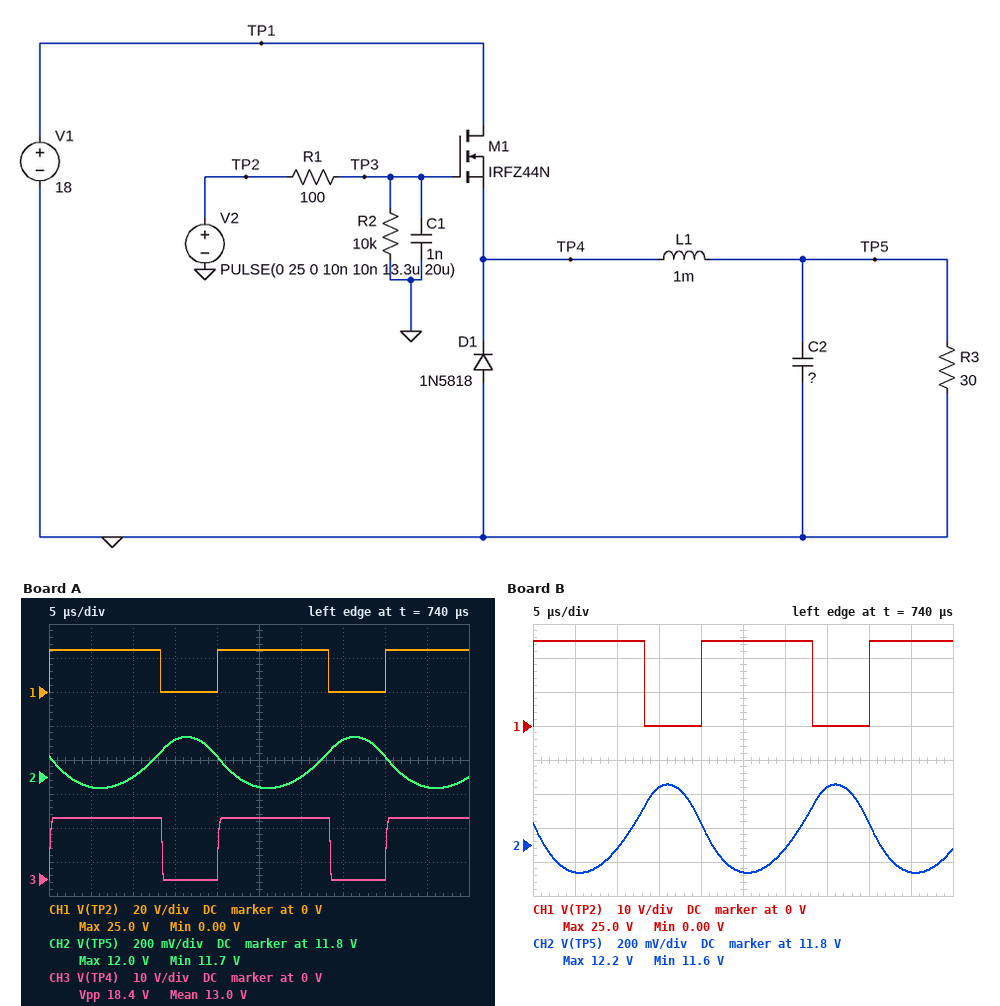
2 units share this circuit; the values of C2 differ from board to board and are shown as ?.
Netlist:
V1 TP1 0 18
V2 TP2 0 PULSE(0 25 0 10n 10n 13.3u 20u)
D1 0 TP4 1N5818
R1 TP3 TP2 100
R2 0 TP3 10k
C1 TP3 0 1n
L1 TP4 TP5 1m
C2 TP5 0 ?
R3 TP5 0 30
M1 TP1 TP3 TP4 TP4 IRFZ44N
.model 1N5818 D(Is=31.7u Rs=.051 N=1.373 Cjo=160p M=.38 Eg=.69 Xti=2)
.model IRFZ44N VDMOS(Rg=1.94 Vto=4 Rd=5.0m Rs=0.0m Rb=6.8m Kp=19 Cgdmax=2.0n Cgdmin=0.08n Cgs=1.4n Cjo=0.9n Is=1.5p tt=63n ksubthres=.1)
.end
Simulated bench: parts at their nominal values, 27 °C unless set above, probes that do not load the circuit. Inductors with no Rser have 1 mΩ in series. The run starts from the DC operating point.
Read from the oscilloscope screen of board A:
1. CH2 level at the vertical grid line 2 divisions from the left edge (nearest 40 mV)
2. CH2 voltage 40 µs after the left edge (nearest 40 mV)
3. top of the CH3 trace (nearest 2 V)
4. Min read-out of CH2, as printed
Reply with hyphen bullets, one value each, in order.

- 11.80 V
- 11.92 V
- 18 V
- 11.7 V
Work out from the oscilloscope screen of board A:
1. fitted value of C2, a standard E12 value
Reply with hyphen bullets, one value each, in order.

- 680 nF
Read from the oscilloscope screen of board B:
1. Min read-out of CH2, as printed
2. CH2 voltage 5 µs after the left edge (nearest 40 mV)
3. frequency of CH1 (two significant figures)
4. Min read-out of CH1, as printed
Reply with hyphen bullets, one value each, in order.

- 11.6 V
- 11.64 V
- 50 kHz
- 0.00 V
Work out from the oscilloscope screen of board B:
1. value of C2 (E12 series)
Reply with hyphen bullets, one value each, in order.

- 390 nF
